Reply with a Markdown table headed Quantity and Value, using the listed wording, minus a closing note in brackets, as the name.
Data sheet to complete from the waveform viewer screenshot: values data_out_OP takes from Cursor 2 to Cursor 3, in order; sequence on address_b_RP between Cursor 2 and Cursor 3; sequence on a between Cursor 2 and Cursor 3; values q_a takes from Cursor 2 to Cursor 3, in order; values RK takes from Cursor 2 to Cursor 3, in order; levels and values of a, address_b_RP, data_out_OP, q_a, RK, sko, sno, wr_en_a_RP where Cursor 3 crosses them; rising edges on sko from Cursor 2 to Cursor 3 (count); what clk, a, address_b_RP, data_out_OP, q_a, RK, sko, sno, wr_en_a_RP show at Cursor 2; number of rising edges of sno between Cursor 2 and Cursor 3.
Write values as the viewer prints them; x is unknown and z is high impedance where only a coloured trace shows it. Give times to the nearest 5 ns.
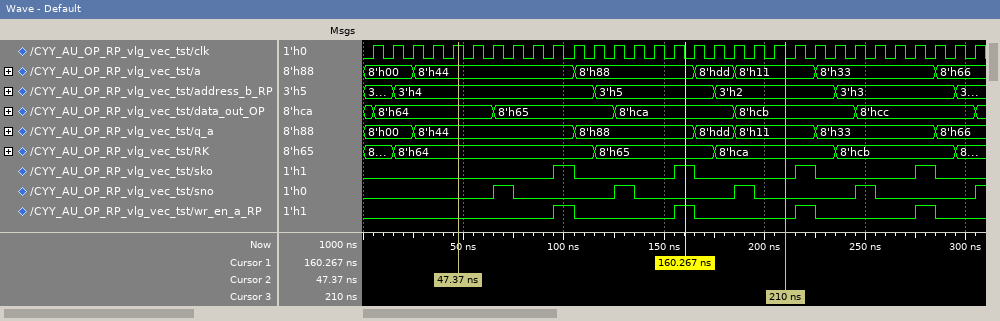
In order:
| Quantity | Value |
|---|---|
| values data_out_OP takes from Cursor 2 to Cursor 3, in order | 8'h64, 8'h65, 8'hca, 8'hcb |
| sequence on address_b_RP between Cursor 2 and Cursor 3 | 3'h4, 3'h5, 3'h2 |
| sequence on a between Cursor 2 and Cursor 3 | 8'h44, 8'h88, 8'hdd, 8'h11 |
| values q_a takes from Cursor 2 to Cursor 3, in order | 8'h44, 8'h88, 8'hdd, 8'h11 |
| values RK takes from Cursor 2 to Cursor 3, in order | 8'h64, 8'h65, 8'hca |
| levels and values of a, address_b_RP, data_out_OP, q_a, RK, sko, sno, wr_en_a_RP where Cursor 3 crosses them | a=8'h11, address_b_RP=3'h2, data_out_OP=8'hcb, q_a=8'h11, RK=8'hca, sko=0, sno=0, wr_en_a_RP=0 |
| rising edges on sko from Cursor 2 to Cursor 3 | 2 |
| what clk, a, address_b_RP, data_out_OP, q_a, RK, sko, sno, wr_en_a_RP show at Cursor 2 | clk=1, a=8'h44, address_b_RP=3'h4, data_out_OP=8'h64, q_a=8'h44, RK=8'h64, sko=0, sno=0, wr_en_a_RP=0 |
| number of rising edges of sno between Cursor 2 and Cursor 3 | 3 |
